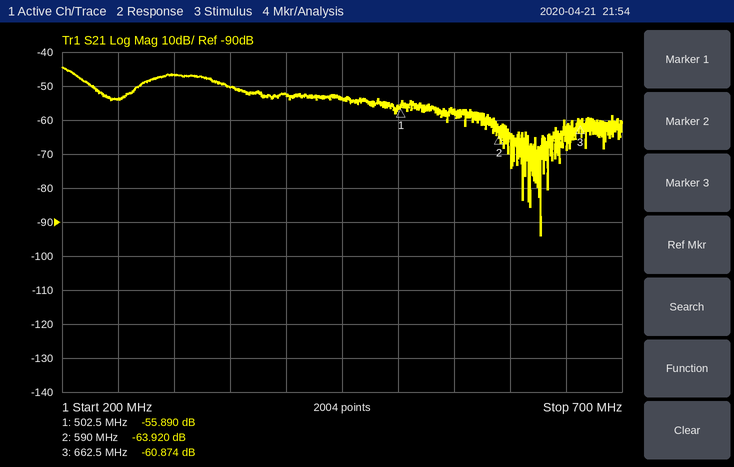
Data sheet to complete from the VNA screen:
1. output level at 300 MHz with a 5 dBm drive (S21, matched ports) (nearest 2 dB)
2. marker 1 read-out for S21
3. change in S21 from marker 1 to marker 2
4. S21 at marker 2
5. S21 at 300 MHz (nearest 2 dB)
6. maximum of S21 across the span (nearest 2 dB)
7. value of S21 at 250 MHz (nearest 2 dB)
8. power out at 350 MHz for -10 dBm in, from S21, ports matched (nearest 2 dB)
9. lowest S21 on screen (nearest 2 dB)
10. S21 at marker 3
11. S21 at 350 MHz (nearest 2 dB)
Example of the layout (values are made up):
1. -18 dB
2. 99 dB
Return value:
1. -42 dBm
2. -55.890 dB
3. -8.030 dB
4. -63.920 dB
5. -46 dB
6. -44 dB
7. -54 dB
8. -60 dBm
9. -94 dB
10. -60.874 dB
11. -50 dB
